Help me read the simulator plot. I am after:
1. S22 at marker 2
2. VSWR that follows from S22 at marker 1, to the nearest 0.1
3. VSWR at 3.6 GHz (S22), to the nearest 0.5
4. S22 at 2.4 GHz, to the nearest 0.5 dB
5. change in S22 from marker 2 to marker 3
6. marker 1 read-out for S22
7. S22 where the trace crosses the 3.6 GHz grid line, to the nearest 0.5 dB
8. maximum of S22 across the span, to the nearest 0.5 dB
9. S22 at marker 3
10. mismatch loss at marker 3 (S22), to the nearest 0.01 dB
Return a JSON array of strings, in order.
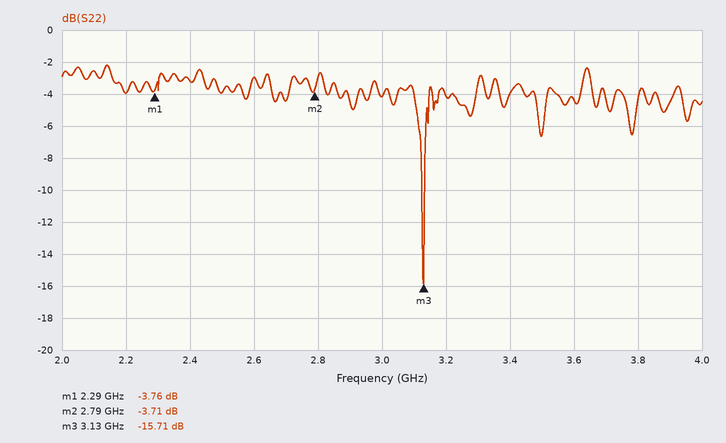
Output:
["-3.71 dB", "4.7", "4.0", "-3.0 dB", "-12.00 dB", "-3.76 dB", "-4.5 dB", "-2.0 dB", "-15.71 dB", "0.12 dB"]
